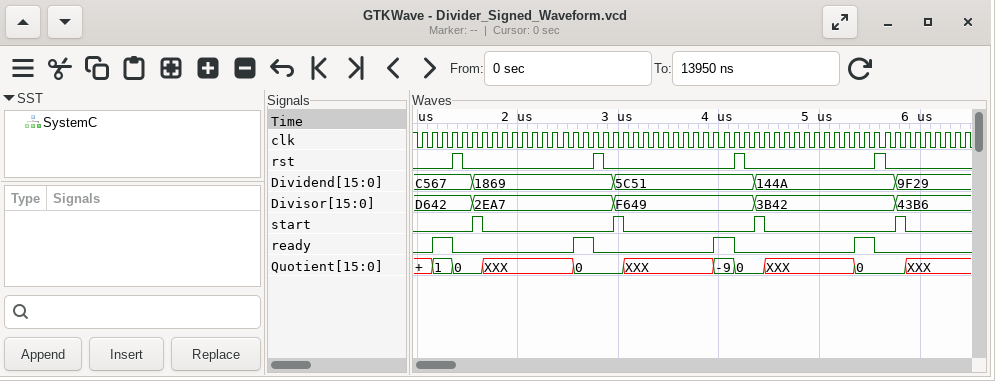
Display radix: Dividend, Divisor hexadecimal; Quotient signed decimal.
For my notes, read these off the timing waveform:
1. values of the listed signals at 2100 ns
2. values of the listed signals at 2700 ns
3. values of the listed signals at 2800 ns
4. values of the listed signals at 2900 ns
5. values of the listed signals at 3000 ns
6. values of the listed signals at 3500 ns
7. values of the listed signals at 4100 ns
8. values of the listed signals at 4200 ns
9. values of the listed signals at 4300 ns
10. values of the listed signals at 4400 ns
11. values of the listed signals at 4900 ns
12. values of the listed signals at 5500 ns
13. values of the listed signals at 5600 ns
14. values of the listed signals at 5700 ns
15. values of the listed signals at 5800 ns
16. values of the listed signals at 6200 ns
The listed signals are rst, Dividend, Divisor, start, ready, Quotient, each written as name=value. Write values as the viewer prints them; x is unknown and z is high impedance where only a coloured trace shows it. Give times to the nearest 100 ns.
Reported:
rst=0, Dividend=1869, Divisor=2EA7, start=0, ready=0, Quotient=XXX
rst=0, Dividend=1869, Divisor=2EA7, start=0, ready=1, Quotient=0
rst=1, Dividend=1869, Divisor=2EA7, start=0, ready=0, Quotient=0
rst=0, Dividend=1869, Divisor=2EA7, start=0, ready=0, Quotient=0
rst=0, Dividend=5C51, Divisor=F649, start=1, ready=0, Quotient=0
rst=0, Dividend=5C51, Divisor=F649, start=0, ready=0, Quotient=XXX
rst=0, Dividend=5C51, Divisor=F649, start=0, ready=1, Quotient=-9
rst=1, Dividend=5C51, Divisor=F649, start=0, ready=0, Quotient=0
rst=0, Dividend=5C51, Divisor=F649, start=0, ready=0, Quotient=0
rst=0, Dividend=144A, Divisor=3B42, start=1, ready=0, Quotient=0
rst=0, Dividend=144A, Divisor=3B42, start=0, ready=0, Quotient=XXX
rst=0, Dividend=144A, Divisor=3B42, start=0, ready=1, Quotient=0
rst=1, Dividend=144A, Divisor=3B42, start=0, ready=0, Quotient=0
rst=0, Dividend=144A, Divisor=3B42, start=0, ready=0, Quotient=0
rst=0, Dividend=9F29, Divisor=43B6, start=1, ready=0, Quotient=0
rst=0, Dividend=9F29, Divisor=43B6, start=0, ready=0, Quotient=XXX
